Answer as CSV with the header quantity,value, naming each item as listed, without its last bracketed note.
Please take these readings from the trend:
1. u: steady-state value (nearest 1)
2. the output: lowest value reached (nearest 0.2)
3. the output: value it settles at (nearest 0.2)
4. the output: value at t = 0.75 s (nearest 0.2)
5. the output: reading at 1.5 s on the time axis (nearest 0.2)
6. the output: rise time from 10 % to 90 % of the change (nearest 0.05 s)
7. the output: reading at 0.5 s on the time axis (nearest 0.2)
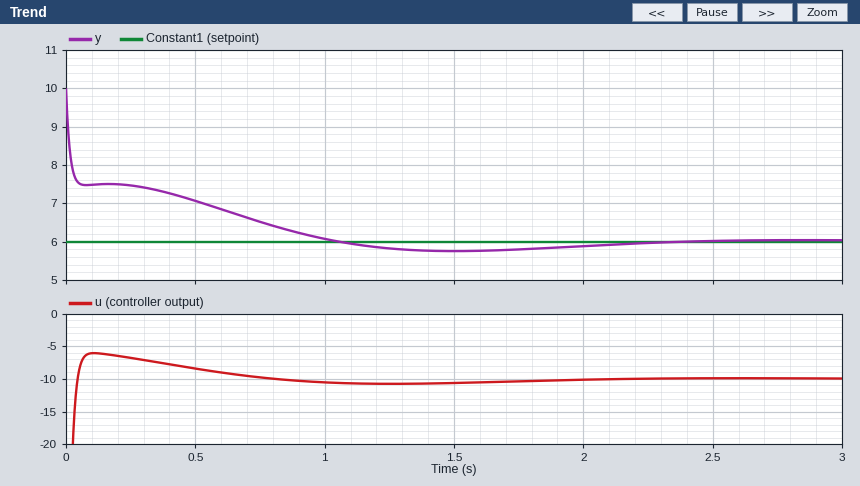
quantity,value
u: steady-state value,-10
the output: lowest value reached,5.8
the output: value it settles at,6.0
the output: value at t = 0.75 s,6.6
the output: reading at 1.5 s on the time axis,5.8
the output: rise time from 10 % to 90 % of the change,0.80 s
the output: reading at 0.5 s on the time axis,7.0
